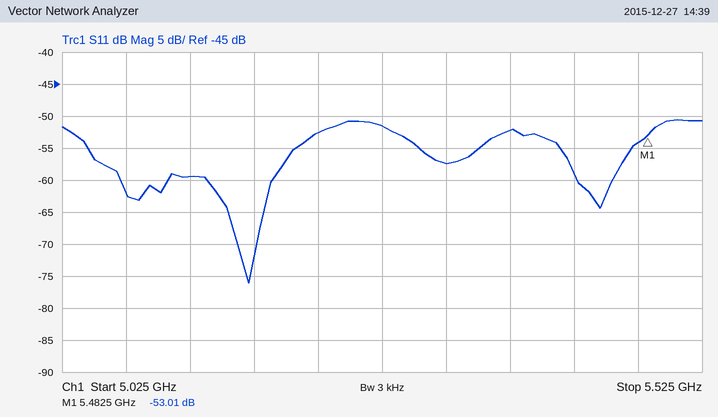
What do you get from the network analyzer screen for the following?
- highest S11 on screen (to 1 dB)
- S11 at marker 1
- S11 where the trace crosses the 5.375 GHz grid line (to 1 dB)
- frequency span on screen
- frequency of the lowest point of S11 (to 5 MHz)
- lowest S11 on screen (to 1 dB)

-51 dB
-53.01 dB
-52 dB
500 MHz
5.170 GHz
-76 dB
